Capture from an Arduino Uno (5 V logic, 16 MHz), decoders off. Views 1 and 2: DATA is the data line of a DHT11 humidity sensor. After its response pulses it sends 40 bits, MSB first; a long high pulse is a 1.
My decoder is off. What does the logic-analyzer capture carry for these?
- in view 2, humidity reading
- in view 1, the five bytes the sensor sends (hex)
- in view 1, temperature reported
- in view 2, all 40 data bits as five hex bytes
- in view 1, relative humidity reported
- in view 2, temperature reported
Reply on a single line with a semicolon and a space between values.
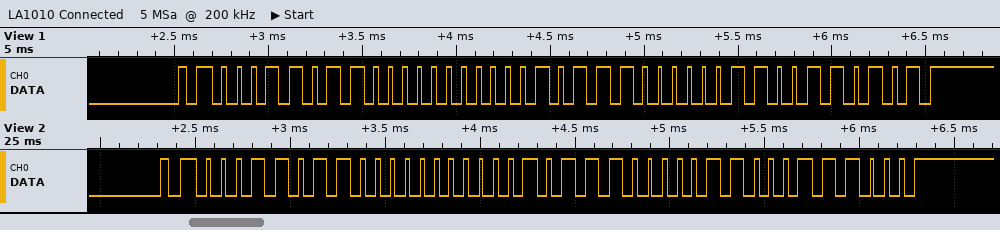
27 %; 1B 00 17 03 35; 23.3 °C; 1B 00 17 06 38; 27 %; 23.6 °C
